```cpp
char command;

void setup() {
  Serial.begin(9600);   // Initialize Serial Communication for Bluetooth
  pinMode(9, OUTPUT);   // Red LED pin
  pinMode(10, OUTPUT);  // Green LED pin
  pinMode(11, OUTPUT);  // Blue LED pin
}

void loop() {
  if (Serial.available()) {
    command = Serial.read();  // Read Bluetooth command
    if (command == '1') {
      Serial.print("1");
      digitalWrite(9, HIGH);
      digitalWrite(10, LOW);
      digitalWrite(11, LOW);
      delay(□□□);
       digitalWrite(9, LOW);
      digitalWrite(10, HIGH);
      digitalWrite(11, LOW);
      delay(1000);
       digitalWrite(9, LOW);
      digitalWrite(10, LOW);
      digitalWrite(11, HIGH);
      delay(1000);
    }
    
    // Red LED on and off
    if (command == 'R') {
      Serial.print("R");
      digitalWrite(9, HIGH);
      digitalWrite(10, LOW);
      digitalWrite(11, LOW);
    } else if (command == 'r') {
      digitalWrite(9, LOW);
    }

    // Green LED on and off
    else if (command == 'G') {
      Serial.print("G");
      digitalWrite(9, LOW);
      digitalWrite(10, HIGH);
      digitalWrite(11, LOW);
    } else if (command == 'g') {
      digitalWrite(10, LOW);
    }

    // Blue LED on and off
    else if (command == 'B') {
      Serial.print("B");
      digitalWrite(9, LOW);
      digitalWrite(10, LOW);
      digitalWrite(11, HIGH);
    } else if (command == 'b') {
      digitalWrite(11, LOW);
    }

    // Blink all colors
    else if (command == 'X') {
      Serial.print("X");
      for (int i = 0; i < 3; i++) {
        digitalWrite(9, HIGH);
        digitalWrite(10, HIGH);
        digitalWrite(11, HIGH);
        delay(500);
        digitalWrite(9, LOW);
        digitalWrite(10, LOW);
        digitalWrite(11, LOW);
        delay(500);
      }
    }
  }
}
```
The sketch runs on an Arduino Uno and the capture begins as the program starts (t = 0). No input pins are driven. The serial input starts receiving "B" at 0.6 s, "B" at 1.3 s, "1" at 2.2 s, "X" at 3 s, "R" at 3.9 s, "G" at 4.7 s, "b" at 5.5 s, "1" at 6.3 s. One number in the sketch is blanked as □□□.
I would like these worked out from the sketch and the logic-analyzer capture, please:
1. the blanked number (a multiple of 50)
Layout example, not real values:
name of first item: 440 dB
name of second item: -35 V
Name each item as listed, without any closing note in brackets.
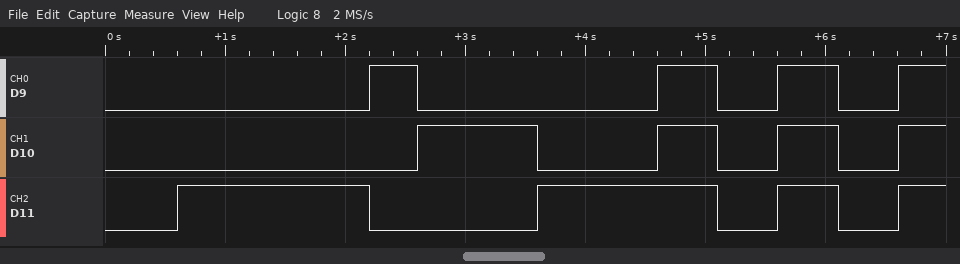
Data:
the blanked number: 400
